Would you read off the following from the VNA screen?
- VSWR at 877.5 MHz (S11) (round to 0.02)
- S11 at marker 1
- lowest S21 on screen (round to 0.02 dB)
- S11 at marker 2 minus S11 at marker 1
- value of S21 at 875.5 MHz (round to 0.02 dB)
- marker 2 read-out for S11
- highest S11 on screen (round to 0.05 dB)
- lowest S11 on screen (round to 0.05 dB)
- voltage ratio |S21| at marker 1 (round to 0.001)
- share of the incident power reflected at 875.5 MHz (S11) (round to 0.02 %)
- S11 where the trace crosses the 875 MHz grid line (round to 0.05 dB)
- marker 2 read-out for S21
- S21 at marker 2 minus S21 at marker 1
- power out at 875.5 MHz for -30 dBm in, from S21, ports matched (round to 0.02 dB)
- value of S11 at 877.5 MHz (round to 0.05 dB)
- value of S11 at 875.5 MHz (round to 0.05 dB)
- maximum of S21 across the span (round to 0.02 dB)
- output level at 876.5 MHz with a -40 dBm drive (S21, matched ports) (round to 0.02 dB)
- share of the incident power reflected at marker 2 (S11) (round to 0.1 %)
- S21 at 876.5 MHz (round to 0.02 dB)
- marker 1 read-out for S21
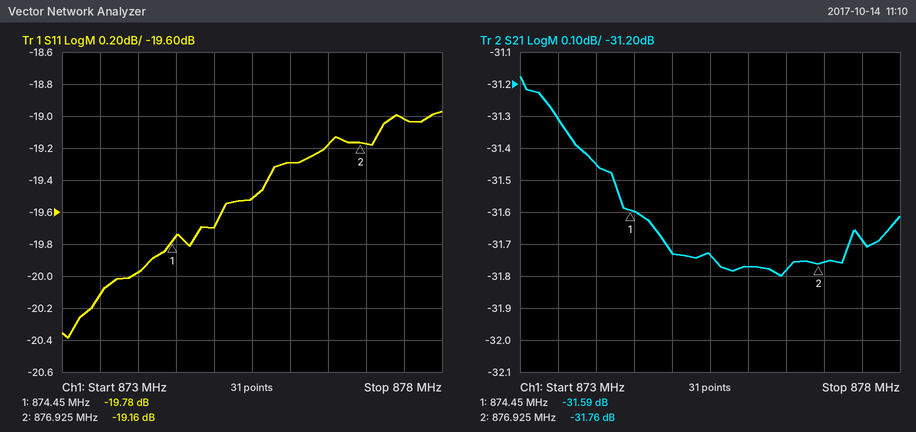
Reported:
1.26
-19.78 dB
-31.80 dB
0.62 dB
-31.74 dB
-19.16 dB
-18.95 dB
-20.40 dB
0.026
1.12 %
-19.70 dB
-31.76 dB
-0.17 dB
-61.74 dBm
-19.00 dB
-19.50 dB
-31.18 dB
-71.78 dBm
1.2 %
-31.78 dB
-31.59 dB
